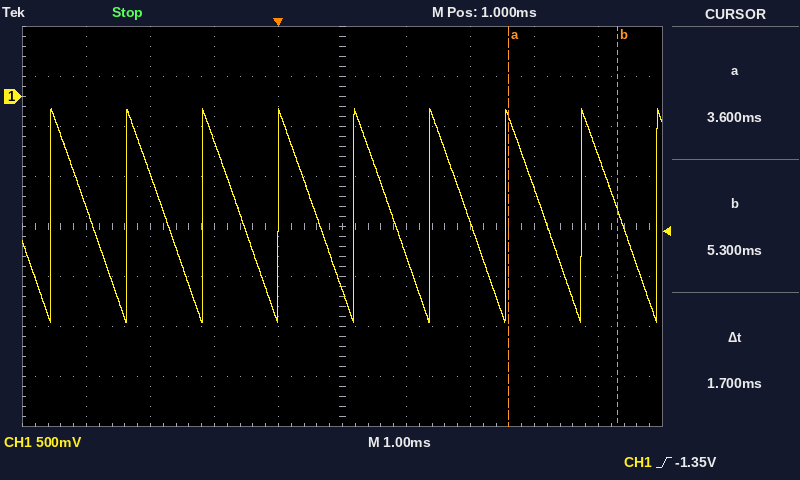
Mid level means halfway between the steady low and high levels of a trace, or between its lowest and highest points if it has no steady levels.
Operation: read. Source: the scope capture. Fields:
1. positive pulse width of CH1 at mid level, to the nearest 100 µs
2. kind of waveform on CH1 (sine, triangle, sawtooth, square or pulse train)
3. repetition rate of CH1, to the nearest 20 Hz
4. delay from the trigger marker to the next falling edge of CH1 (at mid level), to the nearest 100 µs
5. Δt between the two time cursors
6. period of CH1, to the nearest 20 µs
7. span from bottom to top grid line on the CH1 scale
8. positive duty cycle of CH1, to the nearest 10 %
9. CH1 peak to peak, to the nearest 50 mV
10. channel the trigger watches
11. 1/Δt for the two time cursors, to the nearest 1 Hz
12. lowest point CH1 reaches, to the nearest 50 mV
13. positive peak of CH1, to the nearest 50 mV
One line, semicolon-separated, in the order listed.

600 µs; sawtooth; 840 Hz; 600 µs; 1.7 ms; 1.18 ms; 4 V; 50 %; 2.15 V; CH1; 588 Hz; -2.25 V; -100 mV
